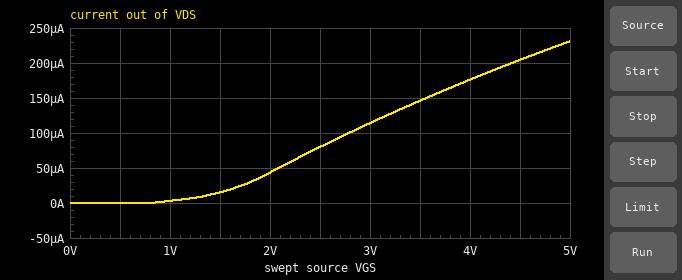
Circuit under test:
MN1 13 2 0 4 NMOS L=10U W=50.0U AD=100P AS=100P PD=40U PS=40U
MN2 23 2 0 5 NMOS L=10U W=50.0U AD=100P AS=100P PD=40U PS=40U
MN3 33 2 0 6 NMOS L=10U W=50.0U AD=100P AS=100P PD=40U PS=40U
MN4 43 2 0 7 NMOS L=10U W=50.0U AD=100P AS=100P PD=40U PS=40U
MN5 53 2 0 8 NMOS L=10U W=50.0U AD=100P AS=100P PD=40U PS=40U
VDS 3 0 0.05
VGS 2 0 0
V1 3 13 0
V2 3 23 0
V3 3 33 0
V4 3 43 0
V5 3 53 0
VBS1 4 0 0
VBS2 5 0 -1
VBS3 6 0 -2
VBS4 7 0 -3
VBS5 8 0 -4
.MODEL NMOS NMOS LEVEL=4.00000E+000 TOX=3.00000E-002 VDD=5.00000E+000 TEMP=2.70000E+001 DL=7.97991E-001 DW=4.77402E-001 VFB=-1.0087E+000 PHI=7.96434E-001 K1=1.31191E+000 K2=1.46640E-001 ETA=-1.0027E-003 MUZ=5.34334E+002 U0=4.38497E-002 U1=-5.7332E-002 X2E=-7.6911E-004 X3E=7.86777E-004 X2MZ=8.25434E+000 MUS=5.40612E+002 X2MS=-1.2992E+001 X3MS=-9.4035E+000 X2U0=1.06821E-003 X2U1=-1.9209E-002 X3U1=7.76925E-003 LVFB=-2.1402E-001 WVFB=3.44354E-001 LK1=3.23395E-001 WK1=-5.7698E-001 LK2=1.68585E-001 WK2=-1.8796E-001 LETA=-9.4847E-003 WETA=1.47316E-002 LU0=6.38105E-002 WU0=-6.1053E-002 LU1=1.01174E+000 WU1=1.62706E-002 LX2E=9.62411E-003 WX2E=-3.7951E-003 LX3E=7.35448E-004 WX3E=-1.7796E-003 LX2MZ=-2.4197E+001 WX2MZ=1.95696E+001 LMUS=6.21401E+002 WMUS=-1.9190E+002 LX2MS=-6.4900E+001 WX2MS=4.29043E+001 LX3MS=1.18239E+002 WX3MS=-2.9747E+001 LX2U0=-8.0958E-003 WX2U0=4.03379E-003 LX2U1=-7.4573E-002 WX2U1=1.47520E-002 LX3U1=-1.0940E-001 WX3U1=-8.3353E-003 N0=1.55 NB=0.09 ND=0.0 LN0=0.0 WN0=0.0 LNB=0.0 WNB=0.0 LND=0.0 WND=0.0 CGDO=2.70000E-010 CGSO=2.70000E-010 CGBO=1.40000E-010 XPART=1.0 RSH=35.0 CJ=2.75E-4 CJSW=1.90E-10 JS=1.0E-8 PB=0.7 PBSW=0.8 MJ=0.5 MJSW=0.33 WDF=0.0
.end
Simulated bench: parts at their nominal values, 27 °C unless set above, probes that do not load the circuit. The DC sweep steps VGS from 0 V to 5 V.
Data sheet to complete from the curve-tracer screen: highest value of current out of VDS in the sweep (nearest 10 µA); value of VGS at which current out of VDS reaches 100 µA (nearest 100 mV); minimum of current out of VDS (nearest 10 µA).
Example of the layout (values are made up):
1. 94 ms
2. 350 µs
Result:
1. 230 µA
2. 2.8 V
3. 0 A
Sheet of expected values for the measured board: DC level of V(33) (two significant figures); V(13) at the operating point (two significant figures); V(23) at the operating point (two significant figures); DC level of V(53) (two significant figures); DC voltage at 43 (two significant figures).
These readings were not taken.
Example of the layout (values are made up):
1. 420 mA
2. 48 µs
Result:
1. 50 mV
2. 50 mV
3. 50 mV
4. 50 mV
5. 50 mV
